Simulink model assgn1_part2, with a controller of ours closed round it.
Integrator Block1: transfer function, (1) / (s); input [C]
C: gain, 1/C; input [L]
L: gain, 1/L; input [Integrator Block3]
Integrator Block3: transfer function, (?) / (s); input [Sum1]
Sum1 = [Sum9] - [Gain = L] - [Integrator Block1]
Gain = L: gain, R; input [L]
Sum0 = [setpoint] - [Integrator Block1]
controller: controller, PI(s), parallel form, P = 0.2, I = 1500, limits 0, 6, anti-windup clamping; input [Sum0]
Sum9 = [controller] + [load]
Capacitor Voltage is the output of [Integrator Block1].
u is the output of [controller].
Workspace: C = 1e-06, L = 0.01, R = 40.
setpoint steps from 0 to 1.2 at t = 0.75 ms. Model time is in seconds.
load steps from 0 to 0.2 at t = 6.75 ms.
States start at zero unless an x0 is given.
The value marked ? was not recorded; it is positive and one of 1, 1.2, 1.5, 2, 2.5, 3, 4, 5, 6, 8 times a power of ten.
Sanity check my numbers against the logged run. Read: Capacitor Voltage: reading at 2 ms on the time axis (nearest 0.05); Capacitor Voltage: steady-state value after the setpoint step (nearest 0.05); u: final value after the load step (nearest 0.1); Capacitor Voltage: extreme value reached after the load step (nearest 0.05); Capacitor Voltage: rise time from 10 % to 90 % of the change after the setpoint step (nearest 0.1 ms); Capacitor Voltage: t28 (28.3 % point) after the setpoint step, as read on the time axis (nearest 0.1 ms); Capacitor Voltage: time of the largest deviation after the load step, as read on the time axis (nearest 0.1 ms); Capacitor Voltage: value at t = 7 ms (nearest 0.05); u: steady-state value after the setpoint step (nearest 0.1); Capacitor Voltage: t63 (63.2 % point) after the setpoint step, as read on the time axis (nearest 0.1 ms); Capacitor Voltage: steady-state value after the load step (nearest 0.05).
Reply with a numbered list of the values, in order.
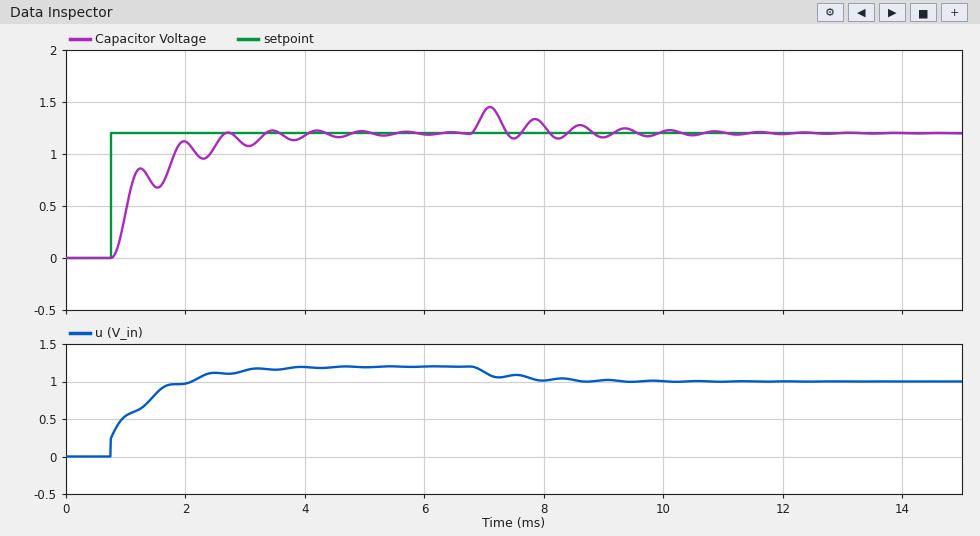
1. 1.10
2. 1.20
3. 1.0
4. 1.45
5. 1.0 ms
6. 1.0 ms
7. 7.1 ms
8. 1.40
9. 1.2
10. 1.1 ms
11. 1.20
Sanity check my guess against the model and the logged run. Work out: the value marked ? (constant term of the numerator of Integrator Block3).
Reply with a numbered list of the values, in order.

1. 0.6
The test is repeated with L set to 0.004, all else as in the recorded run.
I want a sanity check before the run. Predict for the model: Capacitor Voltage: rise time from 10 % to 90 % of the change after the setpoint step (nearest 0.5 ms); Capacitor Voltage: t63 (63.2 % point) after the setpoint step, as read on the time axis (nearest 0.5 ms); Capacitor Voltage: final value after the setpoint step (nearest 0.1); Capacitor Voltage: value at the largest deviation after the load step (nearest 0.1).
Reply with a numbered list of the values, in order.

1. 1.5 ms
2. 1.5 ms
3. 1.2
4. 1.4
